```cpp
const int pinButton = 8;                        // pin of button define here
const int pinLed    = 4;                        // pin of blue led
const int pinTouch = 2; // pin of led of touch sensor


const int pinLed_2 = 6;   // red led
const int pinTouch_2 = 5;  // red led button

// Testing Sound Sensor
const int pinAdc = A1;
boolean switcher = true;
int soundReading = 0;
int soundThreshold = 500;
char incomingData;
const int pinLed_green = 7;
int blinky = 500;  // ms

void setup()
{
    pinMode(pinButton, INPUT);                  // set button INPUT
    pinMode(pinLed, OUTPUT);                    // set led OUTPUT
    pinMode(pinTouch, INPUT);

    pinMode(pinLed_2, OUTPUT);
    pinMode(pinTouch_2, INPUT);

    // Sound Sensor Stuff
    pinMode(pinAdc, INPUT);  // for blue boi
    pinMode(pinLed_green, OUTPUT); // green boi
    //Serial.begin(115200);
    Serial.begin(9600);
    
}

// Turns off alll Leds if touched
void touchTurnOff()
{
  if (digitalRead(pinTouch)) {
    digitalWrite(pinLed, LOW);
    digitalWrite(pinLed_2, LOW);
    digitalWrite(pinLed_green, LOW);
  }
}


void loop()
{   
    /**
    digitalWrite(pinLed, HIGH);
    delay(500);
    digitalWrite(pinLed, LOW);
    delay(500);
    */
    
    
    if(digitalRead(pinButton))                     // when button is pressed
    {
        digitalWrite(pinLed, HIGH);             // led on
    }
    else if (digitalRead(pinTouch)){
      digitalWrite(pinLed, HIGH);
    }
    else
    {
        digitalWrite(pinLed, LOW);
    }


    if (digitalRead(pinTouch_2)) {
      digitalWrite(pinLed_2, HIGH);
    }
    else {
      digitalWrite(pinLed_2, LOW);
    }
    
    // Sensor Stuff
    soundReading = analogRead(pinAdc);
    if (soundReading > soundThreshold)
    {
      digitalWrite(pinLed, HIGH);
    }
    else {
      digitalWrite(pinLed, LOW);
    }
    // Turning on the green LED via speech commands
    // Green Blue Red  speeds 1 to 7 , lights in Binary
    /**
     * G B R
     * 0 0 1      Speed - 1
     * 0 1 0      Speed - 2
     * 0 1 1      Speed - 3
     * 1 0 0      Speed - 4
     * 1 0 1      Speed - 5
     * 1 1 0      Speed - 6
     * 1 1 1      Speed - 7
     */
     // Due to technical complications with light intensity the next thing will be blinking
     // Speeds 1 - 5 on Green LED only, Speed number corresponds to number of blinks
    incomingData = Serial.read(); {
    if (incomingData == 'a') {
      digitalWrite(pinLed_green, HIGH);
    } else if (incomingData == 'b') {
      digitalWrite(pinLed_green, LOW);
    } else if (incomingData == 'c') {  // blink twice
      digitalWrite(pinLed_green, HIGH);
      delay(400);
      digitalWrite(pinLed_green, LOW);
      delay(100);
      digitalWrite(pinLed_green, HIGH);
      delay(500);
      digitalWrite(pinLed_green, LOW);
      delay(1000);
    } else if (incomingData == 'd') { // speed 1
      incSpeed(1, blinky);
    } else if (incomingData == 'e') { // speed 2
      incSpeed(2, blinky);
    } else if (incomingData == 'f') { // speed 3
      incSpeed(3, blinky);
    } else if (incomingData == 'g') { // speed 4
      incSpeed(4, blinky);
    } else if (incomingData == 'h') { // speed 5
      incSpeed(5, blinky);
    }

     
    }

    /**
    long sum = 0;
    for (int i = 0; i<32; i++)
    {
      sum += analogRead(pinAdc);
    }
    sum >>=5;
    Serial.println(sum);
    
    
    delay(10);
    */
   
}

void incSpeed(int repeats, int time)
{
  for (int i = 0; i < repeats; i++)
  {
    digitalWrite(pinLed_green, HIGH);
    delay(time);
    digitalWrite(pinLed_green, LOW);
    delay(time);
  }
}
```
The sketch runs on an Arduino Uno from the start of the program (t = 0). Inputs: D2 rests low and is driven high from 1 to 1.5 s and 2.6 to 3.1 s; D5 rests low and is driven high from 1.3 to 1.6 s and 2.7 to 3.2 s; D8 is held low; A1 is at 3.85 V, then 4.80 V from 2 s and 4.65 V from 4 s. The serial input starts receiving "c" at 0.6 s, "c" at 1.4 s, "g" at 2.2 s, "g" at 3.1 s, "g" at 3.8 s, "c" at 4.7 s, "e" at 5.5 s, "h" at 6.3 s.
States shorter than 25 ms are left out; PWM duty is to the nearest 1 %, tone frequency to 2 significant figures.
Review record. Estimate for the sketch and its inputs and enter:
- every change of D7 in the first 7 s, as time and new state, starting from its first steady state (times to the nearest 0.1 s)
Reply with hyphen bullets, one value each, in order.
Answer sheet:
- 0 s low; 0.6 s high; 1 s low; 1.1 s high; 1.6 s low; 2.6 s high; 3 s low; 3.1 s high; 3.6 s low; 4.6 s high; 5.1 s low; 5.6 s high; 6.1 s low; 6.6 s high
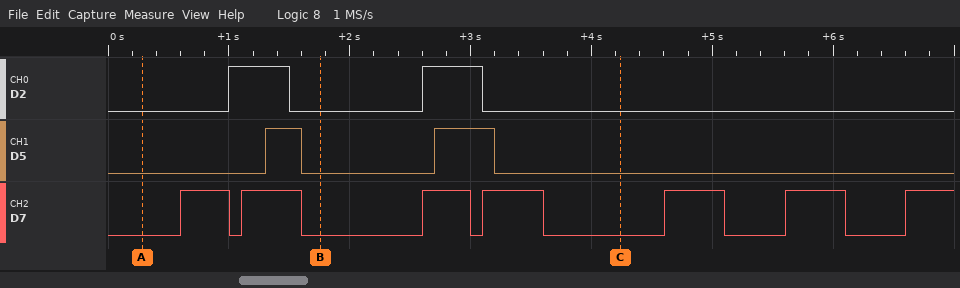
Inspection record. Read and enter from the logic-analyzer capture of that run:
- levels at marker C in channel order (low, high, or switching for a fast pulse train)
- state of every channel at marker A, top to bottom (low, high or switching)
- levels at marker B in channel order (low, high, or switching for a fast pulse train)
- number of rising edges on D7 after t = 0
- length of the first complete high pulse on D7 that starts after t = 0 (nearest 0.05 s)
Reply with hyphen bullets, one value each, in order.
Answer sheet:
- D2 low, D5 low, D7 low
- D2 low, D5 low, D7 low
- D2 low, D5 low, D7 low
- 7
- 0.40 s
